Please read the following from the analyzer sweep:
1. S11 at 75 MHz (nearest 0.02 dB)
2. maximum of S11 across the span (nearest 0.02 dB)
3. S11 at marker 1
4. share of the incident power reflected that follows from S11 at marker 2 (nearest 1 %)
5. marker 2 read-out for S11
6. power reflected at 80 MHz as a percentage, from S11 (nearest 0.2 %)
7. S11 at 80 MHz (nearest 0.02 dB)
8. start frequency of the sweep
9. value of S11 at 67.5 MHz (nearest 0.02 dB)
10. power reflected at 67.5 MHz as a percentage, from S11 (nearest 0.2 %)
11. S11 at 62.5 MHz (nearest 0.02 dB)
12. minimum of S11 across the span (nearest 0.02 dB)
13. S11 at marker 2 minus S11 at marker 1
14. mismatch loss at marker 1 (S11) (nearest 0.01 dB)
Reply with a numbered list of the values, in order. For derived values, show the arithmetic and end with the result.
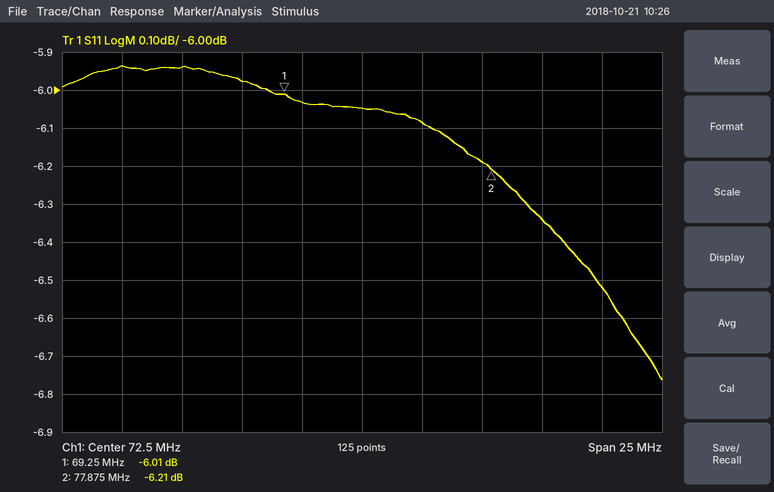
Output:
1. -6.08 dB
2. -5.94 dB
3. -6.01 dB
4. 10^(-6.21/10) ≈ 24 %
5. -6.21 dB
6. 10^(-6.34/10) ≈ 23.2 %
7. -6.34 dB
8. 60 MHz
9. -5.98 dB
10. 10^(-5.98/10) ≈ 25.2 %
11. -5.94 dB
12. -6.76 dB
13. -6.21 − (-6.01) = -0.20 dB
14. −10 log10(1 − 10^(-6.01/10)) ≈ 1.25 dB
